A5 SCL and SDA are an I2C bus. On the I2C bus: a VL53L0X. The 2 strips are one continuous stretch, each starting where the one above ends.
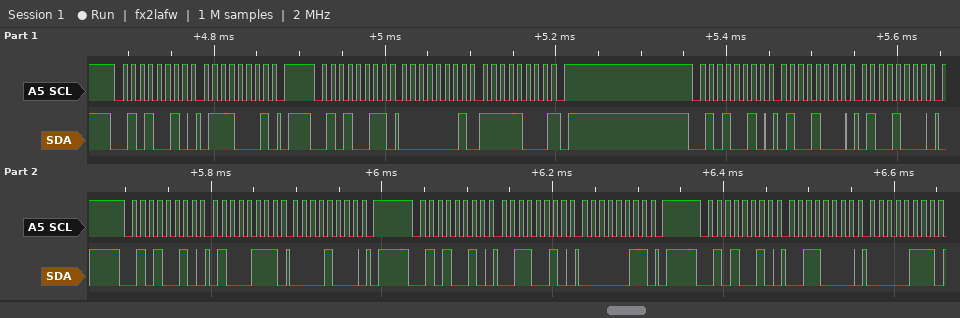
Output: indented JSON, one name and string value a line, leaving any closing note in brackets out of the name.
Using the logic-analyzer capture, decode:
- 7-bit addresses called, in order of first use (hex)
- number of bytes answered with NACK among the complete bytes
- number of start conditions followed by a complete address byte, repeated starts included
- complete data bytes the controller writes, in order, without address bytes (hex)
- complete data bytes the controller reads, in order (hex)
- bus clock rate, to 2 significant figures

{
  "7-bit addresses called, in order of first use": "0x29",
  "number of bytes answered with NACK among the complete bytes": "1",
  "number of start conditions followed by a complete address byte, repeated starts included": "6",
  "complete data bytes the controller writes, in order, without address bytes": "71 48 48 47 08 32 03 30 07",
  "complete data bytes the controller reads, in order": "01 F8",
  "bus clock rate, to 2 significant figures": "100 kHz"
}
